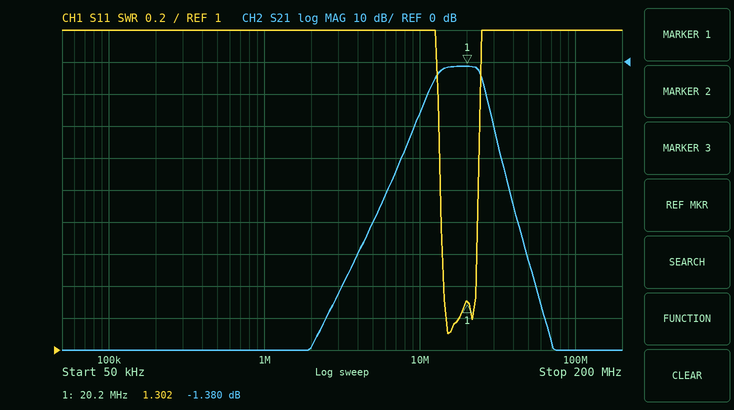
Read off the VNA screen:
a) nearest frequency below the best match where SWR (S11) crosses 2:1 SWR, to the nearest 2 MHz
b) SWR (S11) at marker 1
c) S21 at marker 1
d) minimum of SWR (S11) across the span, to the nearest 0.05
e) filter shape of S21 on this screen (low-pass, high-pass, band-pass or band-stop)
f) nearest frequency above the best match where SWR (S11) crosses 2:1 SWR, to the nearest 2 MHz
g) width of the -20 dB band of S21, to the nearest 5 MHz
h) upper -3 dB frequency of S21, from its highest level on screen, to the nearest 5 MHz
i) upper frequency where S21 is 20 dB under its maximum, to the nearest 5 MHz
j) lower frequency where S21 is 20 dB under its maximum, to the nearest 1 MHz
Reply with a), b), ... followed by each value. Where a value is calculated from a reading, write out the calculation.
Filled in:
a) 14 MHz
b) 1.302
c) -1.380 dB
d) 1.10
e) band-pass
f) 24 MHz
g) 30 MHz − 9 MHz = 21 MHz
h) 25 MHz
i) 30 MHz
j) 9 MHz
